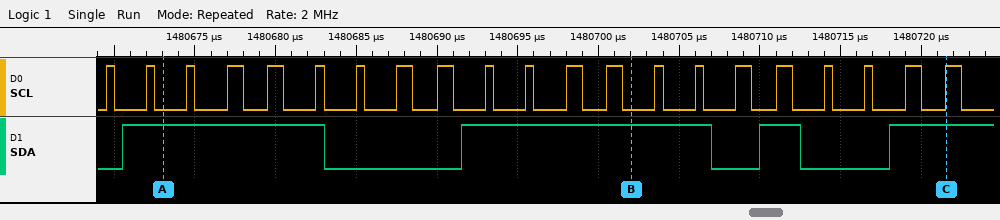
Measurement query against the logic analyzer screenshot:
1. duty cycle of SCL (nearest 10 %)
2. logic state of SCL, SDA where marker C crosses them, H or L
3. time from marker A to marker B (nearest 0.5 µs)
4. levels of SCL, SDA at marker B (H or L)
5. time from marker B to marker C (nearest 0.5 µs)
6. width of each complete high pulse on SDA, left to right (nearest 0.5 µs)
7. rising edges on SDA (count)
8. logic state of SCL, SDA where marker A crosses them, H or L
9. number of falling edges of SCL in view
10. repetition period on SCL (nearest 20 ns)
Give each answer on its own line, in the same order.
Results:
30 %
SCL=H, SDA=H
29 µs
SCL=L, SDA=H
19.5 µs
12.5 µs, 15.5 µs, 2.5 µs
4
SCL=L, SDA=H
21
2600 ns
